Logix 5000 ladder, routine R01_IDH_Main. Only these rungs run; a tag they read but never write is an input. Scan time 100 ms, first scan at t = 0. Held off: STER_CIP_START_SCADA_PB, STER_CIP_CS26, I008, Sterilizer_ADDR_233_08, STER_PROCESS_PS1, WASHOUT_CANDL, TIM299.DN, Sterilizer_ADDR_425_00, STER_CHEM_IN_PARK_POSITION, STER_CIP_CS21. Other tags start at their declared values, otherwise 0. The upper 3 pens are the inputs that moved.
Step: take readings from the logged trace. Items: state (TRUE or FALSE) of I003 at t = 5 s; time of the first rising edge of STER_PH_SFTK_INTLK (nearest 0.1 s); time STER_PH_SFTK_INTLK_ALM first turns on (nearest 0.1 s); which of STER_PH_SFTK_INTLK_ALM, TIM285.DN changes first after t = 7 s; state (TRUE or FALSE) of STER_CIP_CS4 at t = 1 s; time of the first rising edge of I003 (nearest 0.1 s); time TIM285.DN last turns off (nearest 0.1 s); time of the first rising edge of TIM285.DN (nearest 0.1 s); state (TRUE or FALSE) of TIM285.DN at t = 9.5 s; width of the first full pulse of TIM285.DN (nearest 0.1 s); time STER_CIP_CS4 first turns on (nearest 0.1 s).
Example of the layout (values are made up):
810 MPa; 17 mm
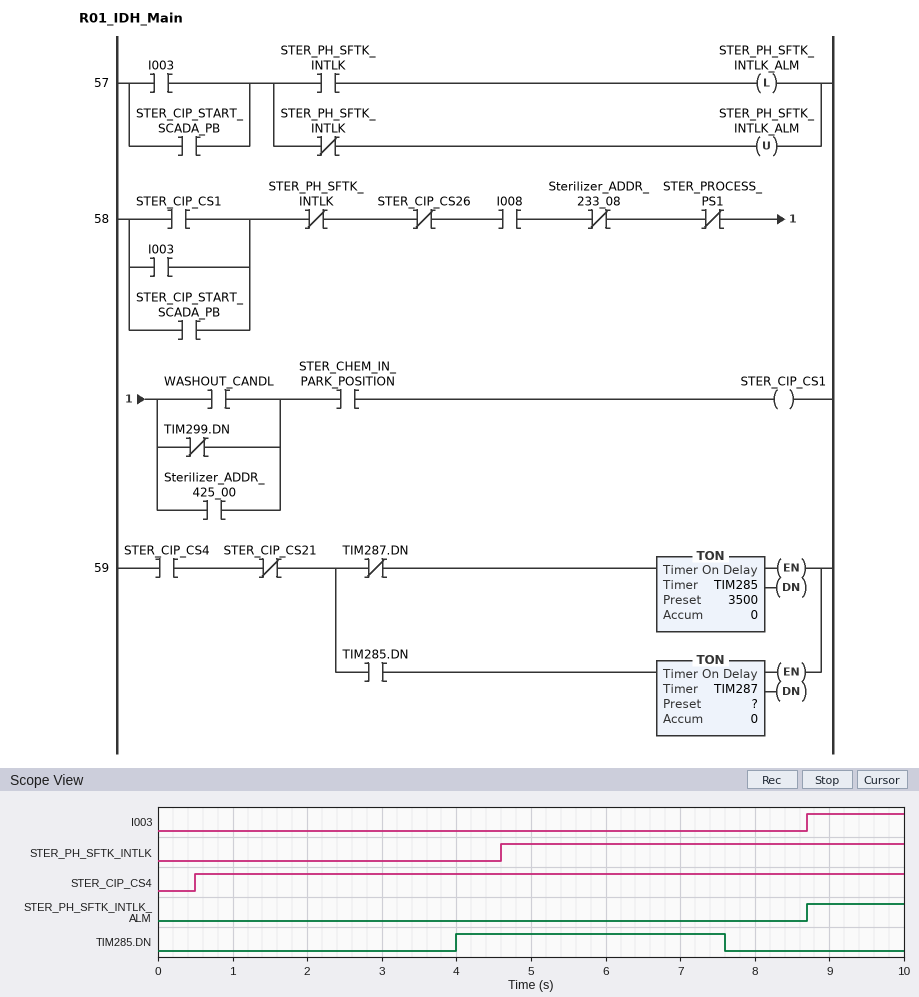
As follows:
FALSE; 4.6 s; 8.7 s; TIM285.DN; TRUE; 8.7 s; 7.6 s; 4.0 s; FALSE; 3.6 s; 0.5 s
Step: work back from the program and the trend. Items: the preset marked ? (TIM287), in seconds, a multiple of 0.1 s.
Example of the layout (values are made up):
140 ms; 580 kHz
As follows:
3.5 s
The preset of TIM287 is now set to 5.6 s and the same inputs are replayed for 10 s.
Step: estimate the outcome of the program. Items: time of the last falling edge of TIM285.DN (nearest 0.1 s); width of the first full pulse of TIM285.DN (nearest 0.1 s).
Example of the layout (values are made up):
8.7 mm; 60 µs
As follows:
9.7 s; 5.7 s
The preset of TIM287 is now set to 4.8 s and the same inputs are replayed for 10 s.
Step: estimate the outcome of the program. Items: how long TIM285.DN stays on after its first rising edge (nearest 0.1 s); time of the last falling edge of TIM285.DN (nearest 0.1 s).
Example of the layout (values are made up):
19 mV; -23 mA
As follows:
4.9 s; 8.9 s
